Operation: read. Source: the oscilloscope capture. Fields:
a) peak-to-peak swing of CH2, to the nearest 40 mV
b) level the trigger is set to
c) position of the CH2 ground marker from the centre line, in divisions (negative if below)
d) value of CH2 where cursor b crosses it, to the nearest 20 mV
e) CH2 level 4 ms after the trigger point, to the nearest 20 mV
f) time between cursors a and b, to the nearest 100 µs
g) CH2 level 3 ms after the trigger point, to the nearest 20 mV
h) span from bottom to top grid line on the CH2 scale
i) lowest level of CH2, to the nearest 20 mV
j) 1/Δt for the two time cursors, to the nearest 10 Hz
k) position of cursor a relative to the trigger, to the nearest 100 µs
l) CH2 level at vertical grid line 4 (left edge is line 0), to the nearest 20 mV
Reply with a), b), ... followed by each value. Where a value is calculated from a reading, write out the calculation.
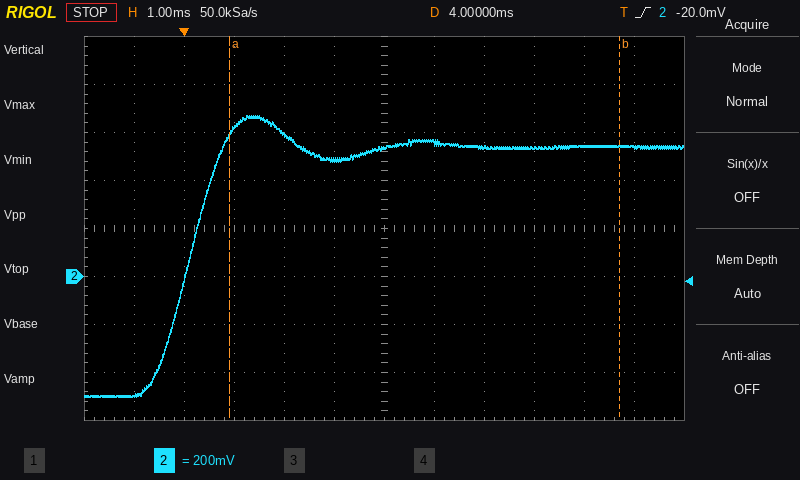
a) 1.16 V
b) -20.0 mV
c) -1.0 div
d) 540 mV
e) 540 mV
f) 7.8 ms
g) 480 mV
h) 1.6 V
i) -500 mV
j) 1 / 7.8 ms ≈ 130 Hz
k) +900 µs
l) 600 mV
